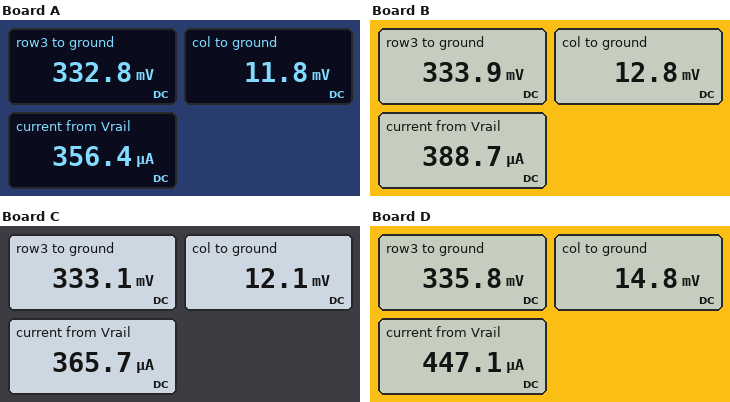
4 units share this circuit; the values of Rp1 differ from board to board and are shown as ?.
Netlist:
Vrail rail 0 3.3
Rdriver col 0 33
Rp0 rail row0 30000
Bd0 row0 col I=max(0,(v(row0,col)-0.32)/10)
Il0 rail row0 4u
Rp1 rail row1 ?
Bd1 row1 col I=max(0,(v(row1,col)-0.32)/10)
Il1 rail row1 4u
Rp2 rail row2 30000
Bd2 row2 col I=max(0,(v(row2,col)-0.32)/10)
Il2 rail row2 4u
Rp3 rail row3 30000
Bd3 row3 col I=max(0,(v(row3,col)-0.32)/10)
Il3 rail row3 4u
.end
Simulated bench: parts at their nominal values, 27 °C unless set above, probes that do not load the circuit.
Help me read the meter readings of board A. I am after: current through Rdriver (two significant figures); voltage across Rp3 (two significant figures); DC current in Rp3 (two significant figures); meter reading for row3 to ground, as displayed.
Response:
360 µA
3.0 V
99 µA
332.8 mV
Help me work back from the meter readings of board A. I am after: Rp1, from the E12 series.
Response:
68 kΩ
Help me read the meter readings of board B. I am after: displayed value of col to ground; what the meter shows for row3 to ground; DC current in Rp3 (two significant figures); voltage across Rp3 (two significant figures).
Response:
12.8 mV
333.9 mV
99 µA
3.0 V
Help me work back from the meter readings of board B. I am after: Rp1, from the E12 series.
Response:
39 kΩ
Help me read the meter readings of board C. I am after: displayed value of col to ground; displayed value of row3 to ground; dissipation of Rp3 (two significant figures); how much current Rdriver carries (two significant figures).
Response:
12.1 mV
333.1 mV
290 µW
370 µA
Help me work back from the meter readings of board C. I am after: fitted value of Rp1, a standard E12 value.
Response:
56 kΩ
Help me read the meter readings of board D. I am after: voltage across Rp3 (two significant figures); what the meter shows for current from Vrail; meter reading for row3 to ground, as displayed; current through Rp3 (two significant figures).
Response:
3.0 V
447.1 µA
335.8 mV
99 µA
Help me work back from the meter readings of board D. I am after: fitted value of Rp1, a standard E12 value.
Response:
22 kΩ
